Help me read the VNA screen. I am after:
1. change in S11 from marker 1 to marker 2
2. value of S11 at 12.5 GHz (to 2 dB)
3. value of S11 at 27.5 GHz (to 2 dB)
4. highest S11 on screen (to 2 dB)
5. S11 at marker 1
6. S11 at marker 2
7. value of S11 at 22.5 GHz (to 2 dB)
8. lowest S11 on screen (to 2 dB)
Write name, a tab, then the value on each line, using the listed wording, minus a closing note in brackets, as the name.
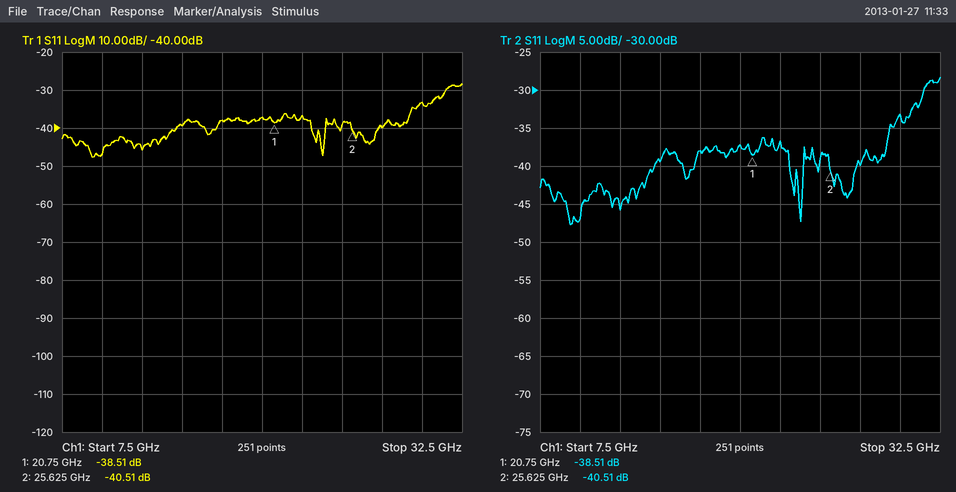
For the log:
change in S11 from marker 1 to marker 2	-2.00 dB
value of S11 at 12.5 GHz	-46 dB
value of S11 at 27.5 GHz	-40 dB
highest S11 on screen	-28 dB
S11 at marker 1	-38.51 dB
S11 at marker 2	-40.51 dB
value of S11 at 22.5 GHz	-36 dB
lowest S11 on screen	-48 dB
